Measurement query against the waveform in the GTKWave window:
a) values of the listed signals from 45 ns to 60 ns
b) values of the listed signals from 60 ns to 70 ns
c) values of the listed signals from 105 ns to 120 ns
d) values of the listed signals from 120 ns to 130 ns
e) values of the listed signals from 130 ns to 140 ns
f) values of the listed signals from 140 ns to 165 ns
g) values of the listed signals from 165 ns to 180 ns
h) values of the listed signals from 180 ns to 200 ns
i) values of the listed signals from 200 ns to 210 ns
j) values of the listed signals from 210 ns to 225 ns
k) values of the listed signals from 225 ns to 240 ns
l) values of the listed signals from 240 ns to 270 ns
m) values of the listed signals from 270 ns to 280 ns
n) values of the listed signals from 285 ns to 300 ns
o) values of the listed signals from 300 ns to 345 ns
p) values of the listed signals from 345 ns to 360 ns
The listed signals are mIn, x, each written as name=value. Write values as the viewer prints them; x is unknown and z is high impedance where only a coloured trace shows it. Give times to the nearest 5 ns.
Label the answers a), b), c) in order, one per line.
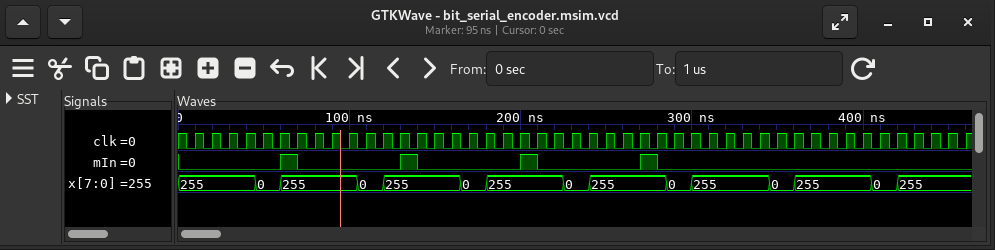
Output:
a) mIn=0, x=0
b) mIn=1, x=255
c) mIn=0, x=0
d) mIn=0, x=255
e) mIn=1, x=255
f) mIn=0, x=255
g) mIn=0, x=0
h) mIn=0, x=255
i) mIn=1, x=255
j) mIn=0, x=255
k) mIn=0, x=0
l) mIn=0, x=255
m) mIn=1, x=255
n) mIn=0, x=0
o) mIn=0, x=255
p) mIn=0, x=0
